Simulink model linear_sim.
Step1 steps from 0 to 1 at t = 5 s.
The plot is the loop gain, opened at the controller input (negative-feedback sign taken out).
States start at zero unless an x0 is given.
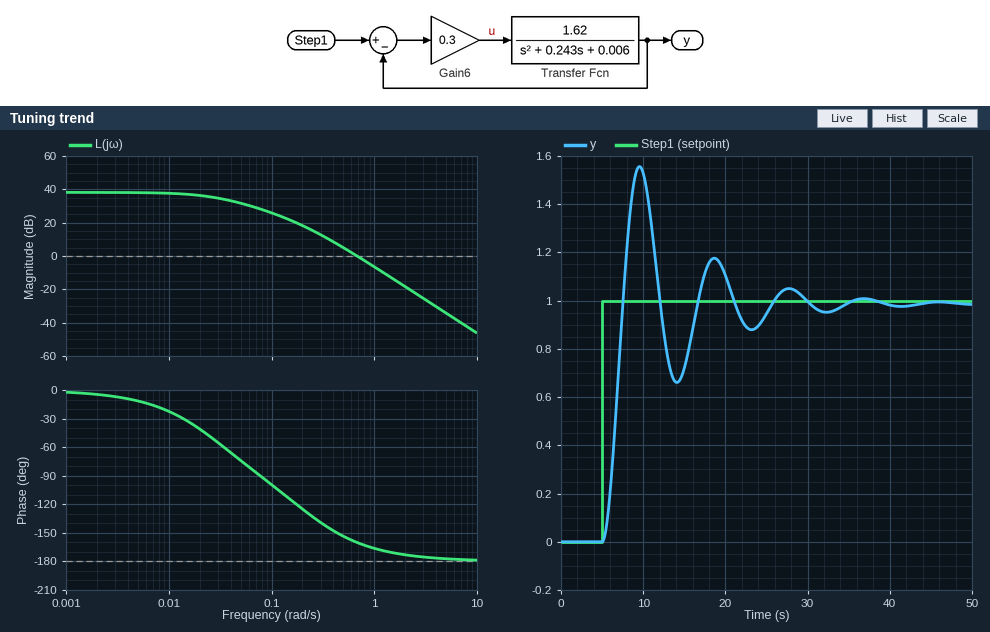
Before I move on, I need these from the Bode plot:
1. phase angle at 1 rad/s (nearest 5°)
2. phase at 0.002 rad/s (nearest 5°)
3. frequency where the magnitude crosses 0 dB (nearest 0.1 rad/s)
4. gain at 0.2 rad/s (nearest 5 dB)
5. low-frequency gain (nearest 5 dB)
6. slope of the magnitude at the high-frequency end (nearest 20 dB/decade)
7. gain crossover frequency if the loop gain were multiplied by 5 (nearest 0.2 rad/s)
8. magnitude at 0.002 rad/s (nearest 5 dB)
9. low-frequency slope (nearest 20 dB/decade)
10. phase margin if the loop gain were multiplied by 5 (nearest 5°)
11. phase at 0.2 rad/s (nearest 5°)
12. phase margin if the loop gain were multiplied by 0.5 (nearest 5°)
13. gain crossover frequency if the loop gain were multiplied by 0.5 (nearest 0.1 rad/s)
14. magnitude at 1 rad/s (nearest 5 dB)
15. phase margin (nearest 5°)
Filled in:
-165°
-5°
0.7 rad/s
20 dB
40 dB
-40 dB/decade
1.6 rad/s
40 dB
0 dB/decade
10°
-125°
30°
0.5 rad/s
-5 dB
20°
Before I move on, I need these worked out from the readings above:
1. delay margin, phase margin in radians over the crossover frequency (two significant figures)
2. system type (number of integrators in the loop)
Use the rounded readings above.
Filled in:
0.50 s
0
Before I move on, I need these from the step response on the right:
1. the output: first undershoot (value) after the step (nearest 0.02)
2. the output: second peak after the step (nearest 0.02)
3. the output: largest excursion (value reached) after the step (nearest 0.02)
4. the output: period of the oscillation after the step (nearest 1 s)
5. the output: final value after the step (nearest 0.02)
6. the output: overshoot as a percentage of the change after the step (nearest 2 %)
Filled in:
0.66
1.18
1.56
9 s
0.98
58 %
